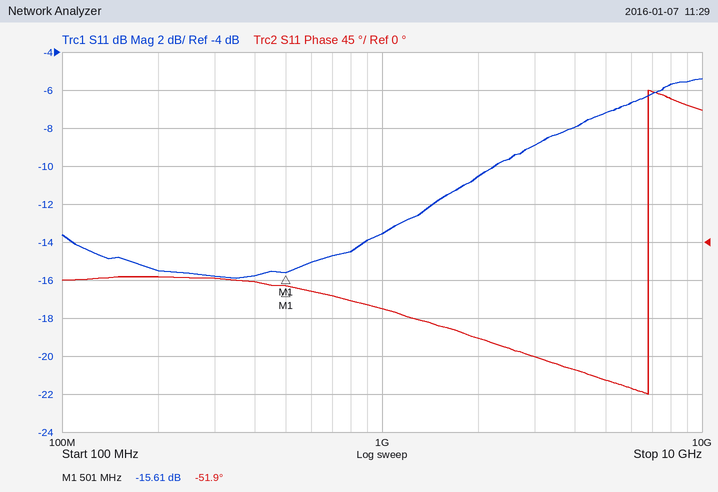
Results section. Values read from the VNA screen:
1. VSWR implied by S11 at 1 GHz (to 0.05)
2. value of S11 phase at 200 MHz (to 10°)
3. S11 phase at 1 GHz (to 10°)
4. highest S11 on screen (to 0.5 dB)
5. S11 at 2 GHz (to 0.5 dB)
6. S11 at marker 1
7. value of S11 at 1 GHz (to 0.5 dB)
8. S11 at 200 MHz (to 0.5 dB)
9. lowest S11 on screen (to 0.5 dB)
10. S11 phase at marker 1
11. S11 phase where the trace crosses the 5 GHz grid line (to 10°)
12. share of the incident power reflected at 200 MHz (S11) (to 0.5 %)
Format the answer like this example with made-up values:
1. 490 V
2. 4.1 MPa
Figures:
1. 1.55
2. -40°
3. -80°
4. -5.5 dB
5. -10.5 dB
6. -15.61 dB
7. -13.5 dB
8. -15.5 dB
9. -16.0 dB
10. -51.9°
11. -160°
12. 3.0 %
